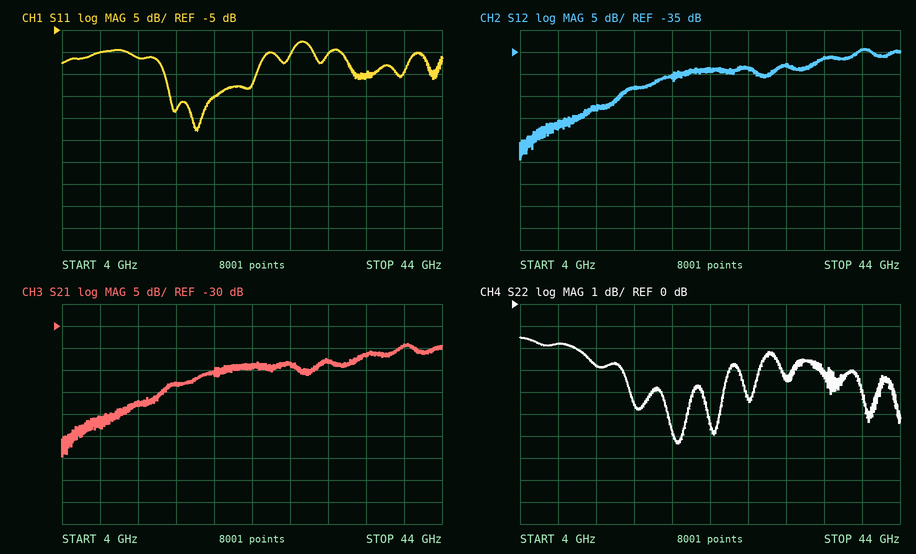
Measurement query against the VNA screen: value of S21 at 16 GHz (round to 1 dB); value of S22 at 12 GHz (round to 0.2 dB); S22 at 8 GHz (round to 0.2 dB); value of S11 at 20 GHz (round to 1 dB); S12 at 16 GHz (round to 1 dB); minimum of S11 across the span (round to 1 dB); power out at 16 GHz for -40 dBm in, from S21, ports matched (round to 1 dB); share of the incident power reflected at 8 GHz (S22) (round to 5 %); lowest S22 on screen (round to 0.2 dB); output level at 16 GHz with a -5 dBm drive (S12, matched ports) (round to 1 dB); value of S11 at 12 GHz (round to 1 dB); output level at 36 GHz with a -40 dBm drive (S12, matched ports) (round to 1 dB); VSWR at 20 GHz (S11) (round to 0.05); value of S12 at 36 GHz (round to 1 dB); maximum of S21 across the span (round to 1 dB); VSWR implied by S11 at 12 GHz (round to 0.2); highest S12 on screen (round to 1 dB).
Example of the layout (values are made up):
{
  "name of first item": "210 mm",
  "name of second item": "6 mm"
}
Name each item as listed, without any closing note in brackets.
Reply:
{
  "value of S21 at 16 GHz": "-43 dB",
  "value of S22 at 12 GHz": "-2.8 dB",
  "S22 at 8 GHz": "-1.8 dB",
  "value of S11 at 20 GHz": "-20 dB",
  "S12 at 16 GHz": "-43 dB",
  "minimum of S11 across the span": "-28 dB",
  "power out at 16 GHz for -40 dBm in, from S21, ports matched": "-83 dBm",
  "share of the incident power reflected at 8 GHz (S22)": "65 %",
  "lowest S22 on screen": "-6.4 dB",
  "output level at 16 GHz with a -5 dBm drive (S12, matched ports)": "-48 dBm",
  "value of S11 at 12 GHz": "-11 dB",
  "output level at 36 GHz with a -40 dBm drive (S12, matched ports)": "-76 dBm",
  "VSWR at 20 GHz (S11)": "1.20",
  "value of S12 at 36 GHz": "-36 dB",
  "maximum of S21 across the span": "-34 dB",
  "VSWR implied by S11 at 12 GHz": "1.8",
  "highest S12 on screen": "-34 dB"
}
